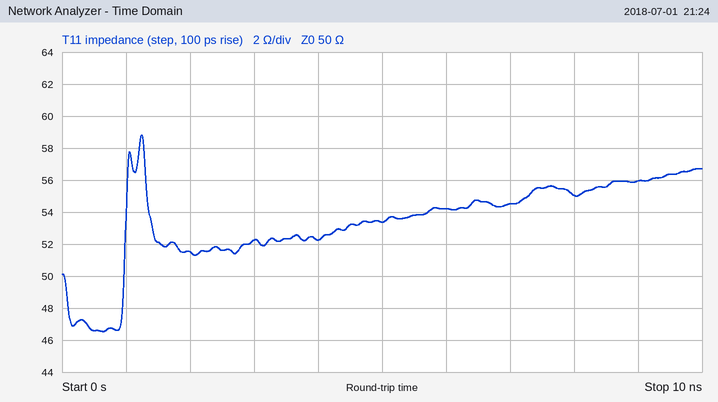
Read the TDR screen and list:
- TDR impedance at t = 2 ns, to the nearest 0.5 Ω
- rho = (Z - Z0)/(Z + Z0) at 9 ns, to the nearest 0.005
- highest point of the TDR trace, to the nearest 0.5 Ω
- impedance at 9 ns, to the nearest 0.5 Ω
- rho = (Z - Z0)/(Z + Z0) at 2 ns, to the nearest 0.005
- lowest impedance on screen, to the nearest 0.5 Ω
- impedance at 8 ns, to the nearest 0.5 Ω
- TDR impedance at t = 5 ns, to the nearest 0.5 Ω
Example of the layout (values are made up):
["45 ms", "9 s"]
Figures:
["51.5 Ω", "+0.055", "59.0 Ω", "56.0 Ω", "+0.015", "46.5 Ω", "55.0 Ω", "53.5 Ω"]
